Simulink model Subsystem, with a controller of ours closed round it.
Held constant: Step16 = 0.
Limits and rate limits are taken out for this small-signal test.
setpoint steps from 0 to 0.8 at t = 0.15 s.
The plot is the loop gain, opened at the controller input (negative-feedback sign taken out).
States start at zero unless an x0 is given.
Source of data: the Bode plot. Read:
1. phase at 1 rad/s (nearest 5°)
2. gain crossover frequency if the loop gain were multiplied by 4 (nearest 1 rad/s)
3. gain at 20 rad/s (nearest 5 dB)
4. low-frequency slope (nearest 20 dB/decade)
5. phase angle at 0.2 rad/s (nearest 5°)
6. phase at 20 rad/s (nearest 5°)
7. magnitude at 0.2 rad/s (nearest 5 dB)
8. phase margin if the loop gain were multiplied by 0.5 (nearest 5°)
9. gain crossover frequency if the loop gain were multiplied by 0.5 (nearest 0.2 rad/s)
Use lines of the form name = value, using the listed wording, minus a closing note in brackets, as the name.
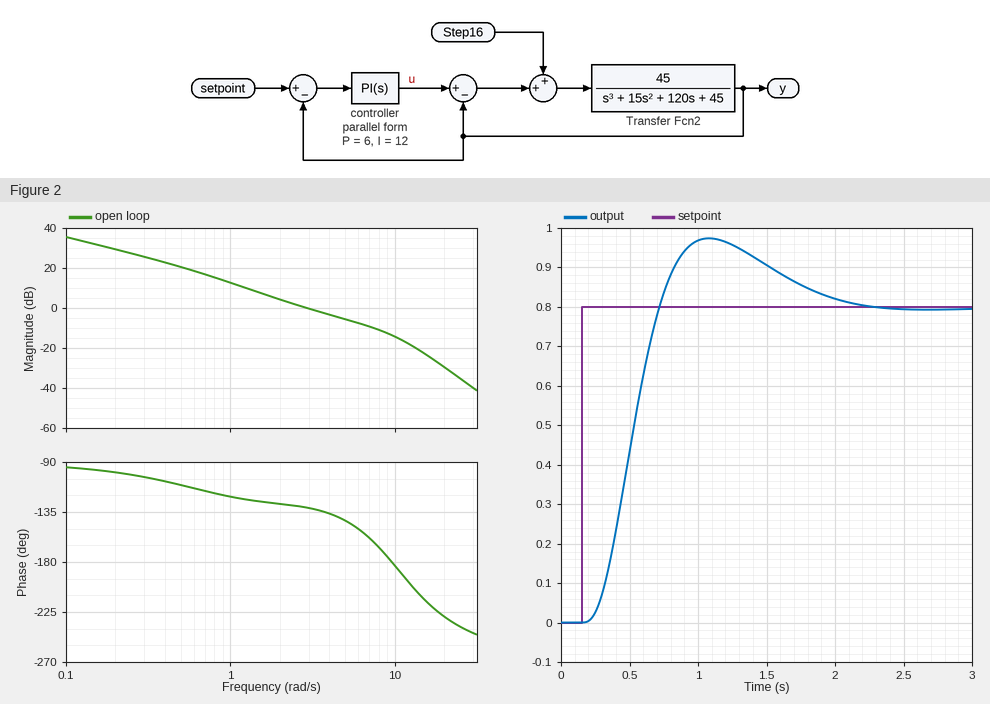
phase at 1 rad/s = -120°
gain crossover frequency if the loop gain were multiplied by 4 = 9 rad/s
gain at 20 rad/s = -30 dB
low-frequency slope = -20 dB/decade
phase angle at 0.2 rad/s = -100°
phase at 20 rad/s = -230°
magnitude at 0.2 rad/s = 30 dB
phase margin if the loop gain were multiplied by 0.5 = 55°
gain crossover frequency if the loop gain were multiplied by 0.5 = 1.8 rad/s
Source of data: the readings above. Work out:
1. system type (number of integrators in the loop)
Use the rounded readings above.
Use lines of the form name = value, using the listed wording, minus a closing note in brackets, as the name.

system type = 1
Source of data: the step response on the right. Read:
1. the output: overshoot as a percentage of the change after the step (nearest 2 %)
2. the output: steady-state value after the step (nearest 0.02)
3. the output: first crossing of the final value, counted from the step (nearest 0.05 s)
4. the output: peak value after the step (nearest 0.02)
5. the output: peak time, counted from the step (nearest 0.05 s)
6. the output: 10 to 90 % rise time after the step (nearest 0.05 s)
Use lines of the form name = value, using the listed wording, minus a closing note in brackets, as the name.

the output: overshoot as a percentage of the change after the step = 22 %
the output: steady-state value after the step = 0.80
the output: first crossing of the final value, counted from the step = 0.55 s
the output: peak value after the step = 0.98
the output: peak time, counted from the step = 0.95 s
the output: 10 to 90 % rise time after the step = 0.35 s
